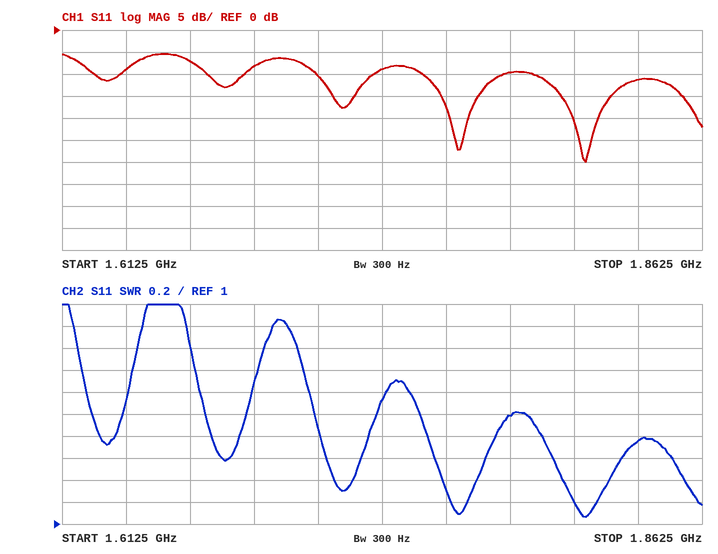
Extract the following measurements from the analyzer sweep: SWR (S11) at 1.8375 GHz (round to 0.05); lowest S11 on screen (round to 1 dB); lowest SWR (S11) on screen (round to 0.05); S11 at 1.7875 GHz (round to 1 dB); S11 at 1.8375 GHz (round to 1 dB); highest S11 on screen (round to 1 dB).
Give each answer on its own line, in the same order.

1.75
-30 dB
1.05
-10 dB
-11 dB
-5 dB
